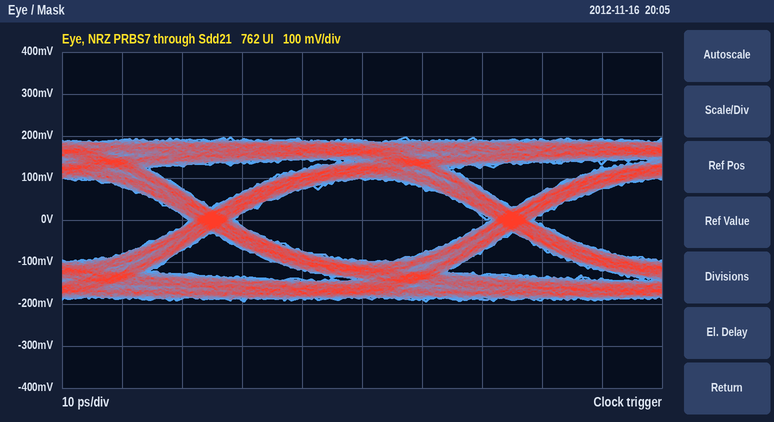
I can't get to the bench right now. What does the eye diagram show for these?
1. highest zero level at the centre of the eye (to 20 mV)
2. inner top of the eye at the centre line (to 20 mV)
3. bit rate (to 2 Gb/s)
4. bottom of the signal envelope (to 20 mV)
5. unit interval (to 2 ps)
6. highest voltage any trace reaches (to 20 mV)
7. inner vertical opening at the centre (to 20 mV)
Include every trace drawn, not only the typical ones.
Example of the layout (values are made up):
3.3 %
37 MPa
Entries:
-100 mV
100 mV
20 Gb/s
-200 mV
50 ps
200 mV
200 mV
